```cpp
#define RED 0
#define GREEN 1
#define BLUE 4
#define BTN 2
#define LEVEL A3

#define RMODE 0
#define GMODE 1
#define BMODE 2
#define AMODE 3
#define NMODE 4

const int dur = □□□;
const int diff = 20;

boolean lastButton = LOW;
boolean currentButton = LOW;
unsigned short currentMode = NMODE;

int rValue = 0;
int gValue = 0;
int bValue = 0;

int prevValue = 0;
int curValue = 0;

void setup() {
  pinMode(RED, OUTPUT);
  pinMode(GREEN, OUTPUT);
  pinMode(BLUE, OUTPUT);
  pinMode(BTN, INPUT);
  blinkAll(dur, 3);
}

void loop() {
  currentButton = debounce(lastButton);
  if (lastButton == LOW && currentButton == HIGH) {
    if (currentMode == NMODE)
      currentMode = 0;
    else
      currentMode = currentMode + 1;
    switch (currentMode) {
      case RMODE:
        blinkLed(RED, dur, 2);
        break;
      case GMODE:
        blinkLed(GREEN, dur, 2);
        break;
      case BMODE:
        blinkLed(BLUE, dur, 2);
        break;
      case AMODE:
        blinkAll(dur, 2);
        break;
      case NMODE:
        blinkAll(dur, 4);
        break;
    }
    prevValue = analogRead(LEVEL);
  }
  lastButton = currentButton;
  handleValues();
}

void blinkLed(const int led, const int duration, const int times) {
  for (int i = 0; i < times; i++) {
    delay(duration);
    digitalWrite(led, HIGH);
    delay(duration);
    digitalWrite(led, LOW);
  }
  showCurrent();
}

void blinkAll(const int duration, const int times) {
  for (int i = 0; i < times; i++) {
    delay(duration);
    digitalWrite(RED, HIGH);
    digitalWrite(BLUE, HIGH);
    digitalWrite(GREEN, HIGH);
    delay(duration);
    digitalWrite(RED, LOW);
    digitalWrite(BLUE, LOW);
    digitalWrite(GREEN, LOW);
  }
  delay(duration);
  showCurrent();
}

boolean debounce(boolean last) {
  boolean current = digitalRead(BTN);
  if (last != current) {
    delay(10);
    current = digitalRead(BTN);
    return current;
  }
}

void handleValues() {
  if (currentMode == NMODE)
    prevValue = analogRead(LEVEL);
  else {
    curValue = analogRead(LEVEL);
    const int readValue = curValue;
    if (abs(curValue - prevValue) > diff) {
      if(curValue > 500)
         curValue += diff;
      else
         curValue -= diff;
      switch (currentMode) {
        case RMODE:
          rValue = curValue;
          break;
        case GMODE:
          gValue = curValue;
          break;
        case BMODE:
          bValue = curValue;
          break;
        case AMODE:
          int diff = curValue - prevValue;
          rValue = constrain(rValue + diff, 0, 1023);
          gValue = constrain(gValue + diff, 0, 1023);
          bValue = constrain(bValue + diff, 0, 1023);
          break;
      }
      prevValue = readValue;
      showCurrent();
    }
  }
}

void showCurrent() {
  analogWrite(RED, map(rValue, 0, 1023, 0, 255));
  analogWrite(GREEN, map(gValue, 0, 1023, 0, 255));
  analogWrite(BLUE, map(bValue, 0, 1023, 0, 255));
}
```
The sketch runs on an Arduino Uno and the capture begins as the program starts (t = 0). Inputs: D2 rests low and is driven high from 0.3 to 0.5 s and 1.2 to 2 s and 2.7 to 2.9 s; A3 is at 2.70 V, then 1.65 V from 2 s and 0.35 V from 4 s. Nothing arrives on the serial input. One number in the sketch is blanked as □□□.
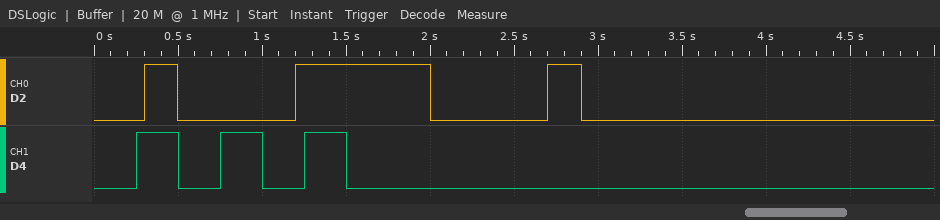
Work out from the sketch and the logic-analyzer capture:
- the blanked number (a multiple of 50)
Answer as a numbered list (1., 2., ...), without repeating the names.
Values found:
1. 250
